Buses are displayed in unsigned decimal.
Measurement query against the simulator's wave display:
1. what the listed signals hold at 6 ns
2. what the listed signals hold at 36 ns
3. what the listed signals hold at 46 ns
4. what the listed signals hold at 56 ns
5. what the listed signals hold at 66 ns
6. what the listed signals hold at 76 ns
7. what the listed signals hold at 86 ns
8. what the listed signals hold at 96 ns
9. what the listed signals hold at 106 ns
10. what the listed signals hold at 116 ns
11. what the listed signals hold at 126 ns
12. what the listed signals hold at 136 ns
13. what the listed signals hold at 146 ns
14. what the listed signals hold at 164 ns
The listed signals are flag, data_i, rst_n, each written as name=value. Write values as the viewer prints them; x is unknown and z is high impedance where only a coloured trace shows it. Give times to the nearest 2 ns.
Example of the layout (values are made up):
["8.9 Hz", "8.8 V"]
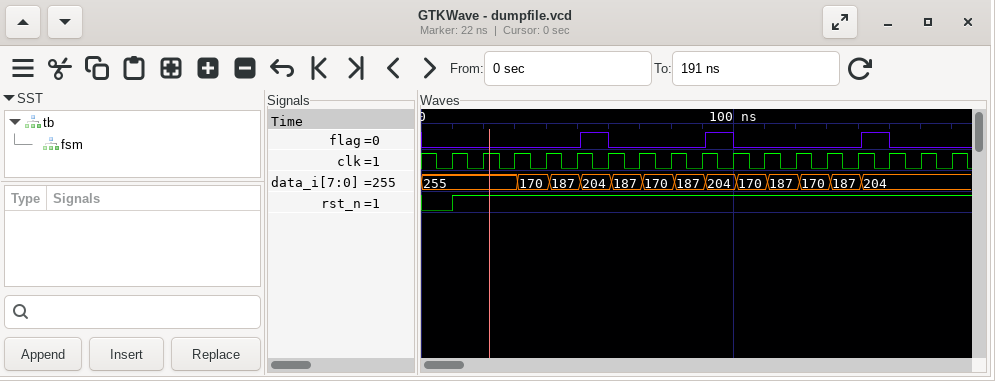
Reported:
["flag=0, data_i=255, rst_n=0", "flag=0, data_i=170, rst_n=1", "flag=0, data_i=187, rst_n=1", "flag=1, data_i=204, rst_n=1", "flag=0, data_i=187, rst_n=1", "flag=0, data_i=170, rst_n=1", "flag=0, data_i=187, rst_n=1", "flag=1, data_i=204, rst_n=1", "flag=0, data_i=170, rst_n=1", "flag=0, data_i=187, rst_n=1", "flag=0, data_i=170, rst_n=1", "flag=0, data_i=187, rst_n=1", "flag=1, data_i=204, rst_n=1", "flag=0, data_i=204, rst_n=1"]
